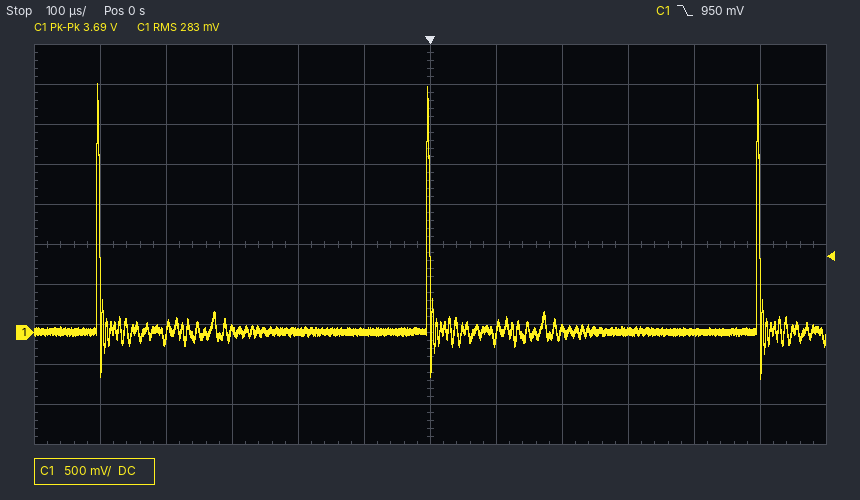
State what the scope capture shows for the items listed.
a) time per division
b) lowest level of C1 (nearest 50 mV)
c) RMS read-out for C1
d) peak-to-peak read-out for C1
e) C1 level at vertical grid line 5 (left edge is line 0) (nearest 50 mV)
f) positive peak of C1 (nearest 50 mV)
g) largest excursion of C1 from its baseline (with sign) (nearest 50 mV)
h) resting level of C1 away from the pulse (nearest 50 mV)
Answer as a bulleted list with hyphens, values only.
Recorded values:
- 100 µs
- -600 mV
- 283 mV
- 3.69 V
- 0 mV
- 3.10 V
- +3.10 V
- 0 mV
